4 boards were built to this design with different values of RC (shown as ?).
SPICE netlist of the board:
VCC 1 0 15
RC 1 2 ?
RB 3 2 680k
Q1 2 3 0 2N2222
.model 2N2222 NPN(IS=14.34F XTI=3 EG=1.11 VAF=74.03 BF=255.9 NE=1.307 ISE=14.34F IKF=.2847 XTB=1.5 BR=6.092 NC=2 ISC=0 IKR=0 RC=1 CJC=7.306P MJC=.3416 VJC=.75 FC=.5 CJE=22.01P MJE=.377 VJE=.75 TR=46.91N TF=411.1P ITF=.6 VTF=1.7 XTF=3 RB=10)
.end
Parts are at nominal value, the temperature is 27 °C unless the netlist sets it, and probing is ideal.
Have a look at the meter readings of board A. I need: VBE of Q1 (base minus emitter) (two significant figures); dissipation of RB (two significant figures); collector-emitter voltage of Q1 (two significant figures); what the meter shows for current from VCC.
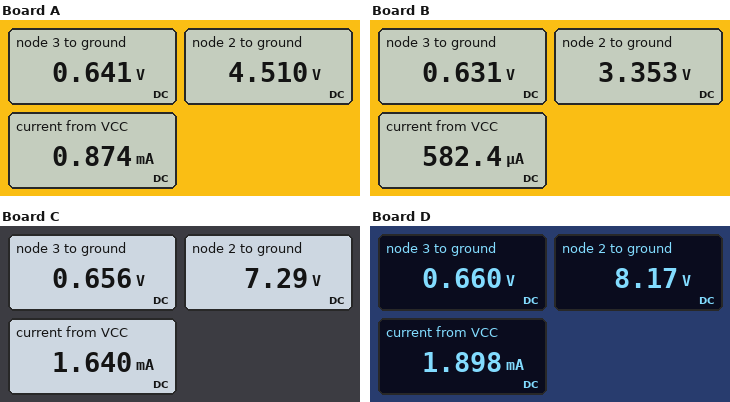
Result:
640 mV
22 µW
4.5 V
0.874 mA
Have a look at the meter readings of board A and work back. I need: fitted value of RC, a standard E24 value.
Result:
12 kΩ
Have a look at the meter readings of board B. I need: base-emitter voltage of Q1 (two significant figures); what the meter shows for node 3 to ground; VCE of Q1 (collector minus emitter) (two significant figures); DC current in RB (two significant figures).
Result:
630 mV
0.631 V
3.4 V
4.0 µA
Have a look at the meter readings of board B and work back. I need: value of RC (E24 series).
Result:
20 kΩ
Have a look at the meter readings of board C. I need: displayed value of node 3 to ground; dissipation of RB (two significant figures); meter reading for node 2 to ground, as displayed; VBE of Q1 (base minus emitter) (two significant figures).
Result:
0.656 V
65 µW
7.29 V
660 mV
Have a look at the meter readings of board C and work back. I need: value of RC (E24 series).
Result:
4.7 kΩ
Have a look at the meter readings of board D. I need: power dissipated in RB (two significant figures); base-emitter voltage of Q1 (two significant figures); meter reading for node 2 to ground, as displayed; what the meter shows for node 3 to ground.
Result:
83 µW
660 mV
8.17 V
0.660 V
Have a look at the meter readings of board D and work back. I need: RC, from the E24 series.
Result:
3.6 kΩ
